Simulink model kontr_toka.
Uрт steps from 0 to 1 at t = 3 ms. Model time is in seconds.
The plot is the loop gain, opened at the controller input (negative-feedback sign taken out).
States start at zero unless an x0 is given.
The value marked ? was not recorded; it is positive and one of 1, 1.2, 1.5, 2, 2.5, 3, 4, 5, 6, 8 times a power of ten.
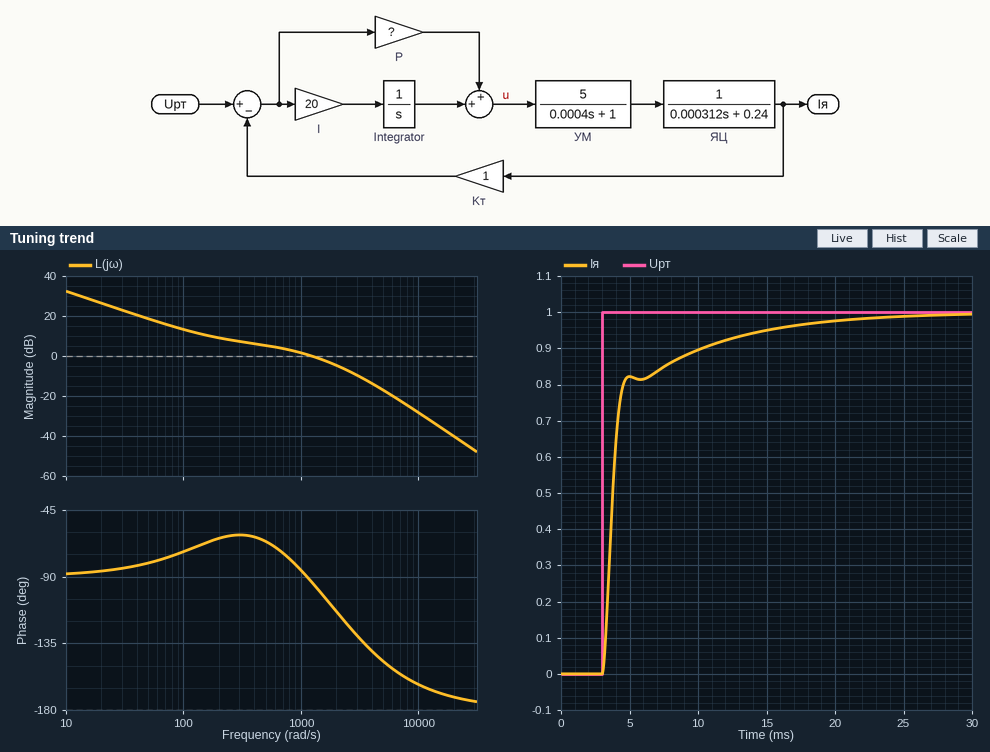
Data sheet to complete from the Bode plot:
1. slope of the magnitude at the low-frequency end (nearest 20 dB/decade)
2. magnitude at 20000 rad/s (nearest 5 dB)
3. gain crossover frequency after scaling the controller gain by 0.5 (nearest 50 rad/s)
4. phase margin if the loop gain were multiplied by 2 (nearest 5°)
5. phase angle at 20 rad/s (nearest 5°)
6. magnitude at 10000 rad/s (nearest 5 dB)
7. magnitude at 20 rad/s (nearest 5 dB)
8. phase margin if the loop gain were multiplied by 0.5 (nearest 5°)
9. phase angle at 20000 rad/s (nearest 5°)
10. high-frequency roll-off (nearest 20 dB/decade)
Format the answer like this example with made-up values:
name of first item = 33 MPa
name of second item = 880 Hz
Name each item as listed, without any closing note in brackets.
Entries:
slope of the magnitude at the low-frequency end = -20 dB/decade
magnitude at 20000 rad/s = -40 dB
gain crossover frequency after scaling the controller gain by 0.5 = 400 rad/s
phase margin if the loop gain were multiplied by 2 = 60°
phase angle at 20 rad/s = -85°
magnitude at 10000 rad/s = -30 dB
magnitude at 20 rad/s = 25 dB
phase margin if the loop gain were multiplied by 0.5 = 115°
phase angle at 20000 rad/s = -170°
high-frequency roll-off = -40 dB/decade
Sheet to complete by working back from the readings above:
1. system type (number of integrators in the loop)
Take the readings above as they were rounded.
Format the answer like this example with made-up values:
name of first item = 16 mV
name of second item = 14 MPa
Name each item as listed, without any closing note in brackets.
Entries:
system type = 1
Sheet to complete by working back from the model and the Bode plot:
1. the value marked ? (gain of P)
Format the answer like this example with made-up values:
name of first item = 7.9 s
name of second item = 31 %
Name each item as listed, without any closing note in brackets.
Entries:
the value marked ? = 0.1
